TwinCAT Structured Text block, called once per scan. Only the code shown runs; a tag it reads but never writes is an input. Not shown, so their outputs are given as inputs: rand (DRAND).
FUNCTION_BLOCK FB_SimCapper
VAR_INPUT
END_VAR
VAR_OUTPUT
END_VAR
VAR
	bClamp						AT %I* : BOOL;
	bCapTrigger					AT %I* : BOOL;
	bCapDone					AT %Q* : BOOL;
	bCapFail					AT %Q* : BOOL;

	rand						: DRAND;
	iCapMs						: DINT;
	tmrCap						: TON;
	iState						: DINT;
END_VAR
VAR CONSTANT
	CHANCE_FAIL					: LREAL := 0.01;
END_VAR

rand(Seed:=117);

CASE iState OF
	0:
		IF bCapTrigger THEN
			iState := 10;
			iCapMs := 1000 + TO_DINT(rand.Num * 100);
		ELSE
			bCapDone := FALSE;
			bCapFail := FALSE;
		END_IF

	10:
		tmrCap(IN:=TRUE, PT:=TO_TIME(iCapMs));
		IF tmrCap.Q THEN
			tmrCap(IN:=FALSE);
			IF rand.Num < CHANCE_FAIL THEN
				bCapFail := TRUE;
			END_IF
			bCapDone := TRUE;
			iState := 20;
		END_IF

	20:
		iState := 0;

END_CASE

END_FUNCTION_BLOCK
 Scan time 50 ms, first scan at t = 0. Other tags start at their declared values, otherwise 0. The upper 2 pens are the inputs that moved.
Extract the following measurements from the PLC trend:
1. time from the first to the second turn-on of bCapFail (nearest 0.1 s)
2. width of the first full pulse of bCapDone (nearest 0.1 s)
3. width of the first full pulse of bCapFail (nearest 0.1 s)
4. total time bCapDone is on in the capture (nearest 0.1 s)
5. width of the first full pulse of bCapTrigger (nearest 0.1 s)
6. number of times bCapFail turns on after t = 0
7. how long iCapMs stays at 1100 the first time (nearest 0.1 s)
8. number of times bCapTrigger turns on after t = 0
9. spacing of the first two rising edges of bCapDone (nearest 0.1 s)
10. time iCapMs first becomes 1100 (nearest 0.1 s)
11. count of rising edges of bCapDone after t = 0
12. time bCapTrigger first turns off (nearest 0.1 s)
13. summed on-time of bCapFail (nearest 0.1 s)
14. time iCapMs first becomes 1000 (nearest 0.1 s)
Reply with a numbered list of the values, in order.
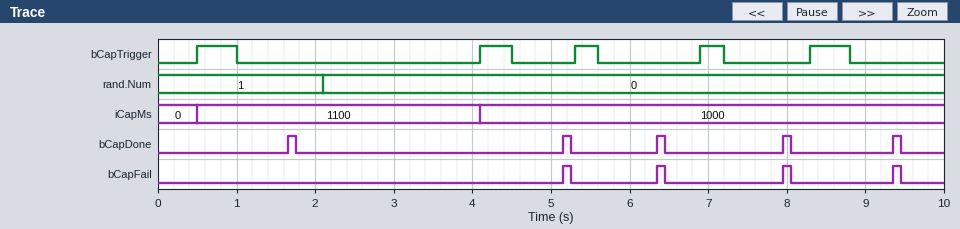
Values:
1. 1.2 s
2. 0.1 s
3. 0.1 s
4. 0.5 s
5. 0.5 s
6. 4
7. 3.6 s
8. 5
9. 3.5 s
10. 0.5 s
11. 5
12. 1.0 s
13. 0.4 s
14. 4.1 s
